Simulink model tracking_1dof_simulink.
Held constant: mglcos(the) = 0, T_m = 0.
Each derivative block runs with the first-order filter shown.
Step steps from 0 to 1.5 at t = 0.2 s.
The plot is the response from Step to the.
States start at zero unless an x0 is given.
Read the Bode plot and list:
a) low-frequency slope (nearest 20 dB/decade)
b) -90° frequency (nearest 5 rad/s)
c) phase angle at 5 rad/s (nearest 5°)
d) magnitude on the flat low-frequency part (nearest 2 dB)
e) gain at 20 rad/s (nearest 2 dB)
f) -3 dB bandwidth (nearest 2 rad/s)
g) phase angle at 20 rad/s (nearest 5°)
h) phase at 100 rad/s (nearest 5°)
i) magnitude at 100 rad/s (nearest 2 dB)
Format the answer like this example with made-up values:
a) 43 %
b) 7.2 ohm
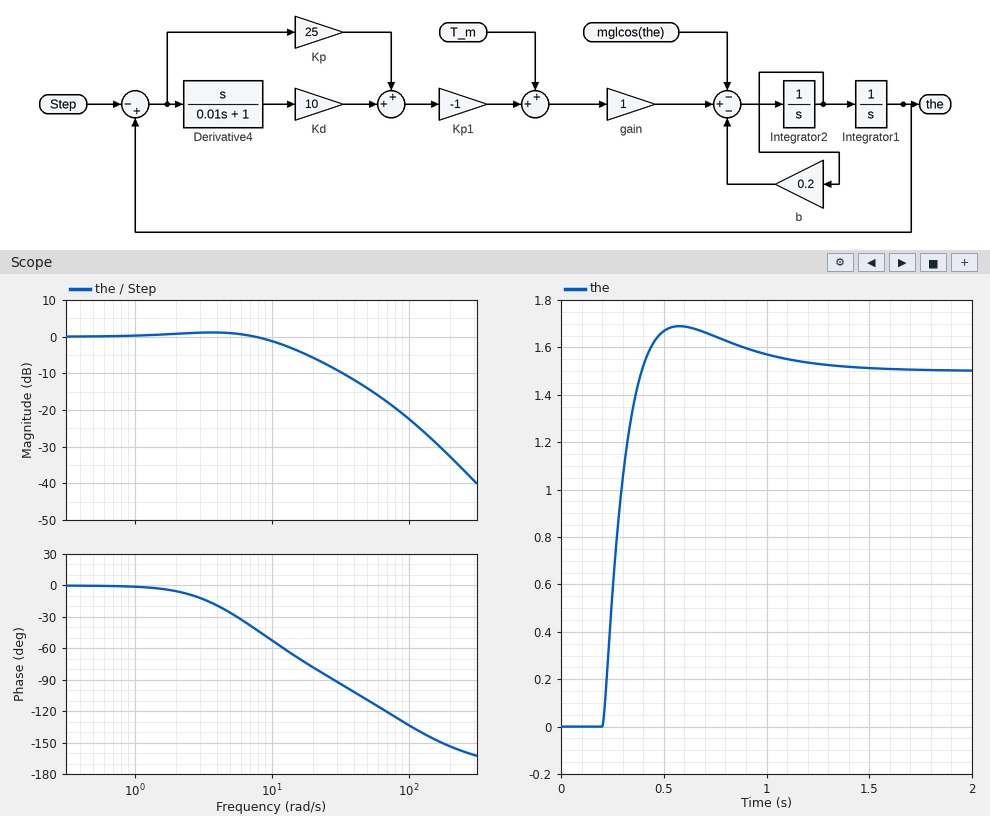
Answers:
a) 0 dB/decade
b) 30 rad/s
c) -25°
d) 0 dB
e) -6 dB
f) 14 rad/s
g) -80°
h) -135°
i) -22 dB
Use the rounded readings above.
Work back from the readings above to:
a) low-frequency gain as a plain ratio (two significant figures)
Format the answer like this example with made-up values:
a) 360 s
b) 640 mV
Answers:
a) 1.0
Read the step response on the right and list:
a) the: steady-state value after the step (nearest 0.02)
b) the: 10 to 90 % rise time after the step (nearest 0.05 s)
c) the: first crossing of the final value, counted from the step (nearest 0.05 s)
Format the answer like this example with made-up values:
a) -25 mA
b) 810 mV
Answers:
a) 1.50
b) 0.15 s
c) 0.20 s
